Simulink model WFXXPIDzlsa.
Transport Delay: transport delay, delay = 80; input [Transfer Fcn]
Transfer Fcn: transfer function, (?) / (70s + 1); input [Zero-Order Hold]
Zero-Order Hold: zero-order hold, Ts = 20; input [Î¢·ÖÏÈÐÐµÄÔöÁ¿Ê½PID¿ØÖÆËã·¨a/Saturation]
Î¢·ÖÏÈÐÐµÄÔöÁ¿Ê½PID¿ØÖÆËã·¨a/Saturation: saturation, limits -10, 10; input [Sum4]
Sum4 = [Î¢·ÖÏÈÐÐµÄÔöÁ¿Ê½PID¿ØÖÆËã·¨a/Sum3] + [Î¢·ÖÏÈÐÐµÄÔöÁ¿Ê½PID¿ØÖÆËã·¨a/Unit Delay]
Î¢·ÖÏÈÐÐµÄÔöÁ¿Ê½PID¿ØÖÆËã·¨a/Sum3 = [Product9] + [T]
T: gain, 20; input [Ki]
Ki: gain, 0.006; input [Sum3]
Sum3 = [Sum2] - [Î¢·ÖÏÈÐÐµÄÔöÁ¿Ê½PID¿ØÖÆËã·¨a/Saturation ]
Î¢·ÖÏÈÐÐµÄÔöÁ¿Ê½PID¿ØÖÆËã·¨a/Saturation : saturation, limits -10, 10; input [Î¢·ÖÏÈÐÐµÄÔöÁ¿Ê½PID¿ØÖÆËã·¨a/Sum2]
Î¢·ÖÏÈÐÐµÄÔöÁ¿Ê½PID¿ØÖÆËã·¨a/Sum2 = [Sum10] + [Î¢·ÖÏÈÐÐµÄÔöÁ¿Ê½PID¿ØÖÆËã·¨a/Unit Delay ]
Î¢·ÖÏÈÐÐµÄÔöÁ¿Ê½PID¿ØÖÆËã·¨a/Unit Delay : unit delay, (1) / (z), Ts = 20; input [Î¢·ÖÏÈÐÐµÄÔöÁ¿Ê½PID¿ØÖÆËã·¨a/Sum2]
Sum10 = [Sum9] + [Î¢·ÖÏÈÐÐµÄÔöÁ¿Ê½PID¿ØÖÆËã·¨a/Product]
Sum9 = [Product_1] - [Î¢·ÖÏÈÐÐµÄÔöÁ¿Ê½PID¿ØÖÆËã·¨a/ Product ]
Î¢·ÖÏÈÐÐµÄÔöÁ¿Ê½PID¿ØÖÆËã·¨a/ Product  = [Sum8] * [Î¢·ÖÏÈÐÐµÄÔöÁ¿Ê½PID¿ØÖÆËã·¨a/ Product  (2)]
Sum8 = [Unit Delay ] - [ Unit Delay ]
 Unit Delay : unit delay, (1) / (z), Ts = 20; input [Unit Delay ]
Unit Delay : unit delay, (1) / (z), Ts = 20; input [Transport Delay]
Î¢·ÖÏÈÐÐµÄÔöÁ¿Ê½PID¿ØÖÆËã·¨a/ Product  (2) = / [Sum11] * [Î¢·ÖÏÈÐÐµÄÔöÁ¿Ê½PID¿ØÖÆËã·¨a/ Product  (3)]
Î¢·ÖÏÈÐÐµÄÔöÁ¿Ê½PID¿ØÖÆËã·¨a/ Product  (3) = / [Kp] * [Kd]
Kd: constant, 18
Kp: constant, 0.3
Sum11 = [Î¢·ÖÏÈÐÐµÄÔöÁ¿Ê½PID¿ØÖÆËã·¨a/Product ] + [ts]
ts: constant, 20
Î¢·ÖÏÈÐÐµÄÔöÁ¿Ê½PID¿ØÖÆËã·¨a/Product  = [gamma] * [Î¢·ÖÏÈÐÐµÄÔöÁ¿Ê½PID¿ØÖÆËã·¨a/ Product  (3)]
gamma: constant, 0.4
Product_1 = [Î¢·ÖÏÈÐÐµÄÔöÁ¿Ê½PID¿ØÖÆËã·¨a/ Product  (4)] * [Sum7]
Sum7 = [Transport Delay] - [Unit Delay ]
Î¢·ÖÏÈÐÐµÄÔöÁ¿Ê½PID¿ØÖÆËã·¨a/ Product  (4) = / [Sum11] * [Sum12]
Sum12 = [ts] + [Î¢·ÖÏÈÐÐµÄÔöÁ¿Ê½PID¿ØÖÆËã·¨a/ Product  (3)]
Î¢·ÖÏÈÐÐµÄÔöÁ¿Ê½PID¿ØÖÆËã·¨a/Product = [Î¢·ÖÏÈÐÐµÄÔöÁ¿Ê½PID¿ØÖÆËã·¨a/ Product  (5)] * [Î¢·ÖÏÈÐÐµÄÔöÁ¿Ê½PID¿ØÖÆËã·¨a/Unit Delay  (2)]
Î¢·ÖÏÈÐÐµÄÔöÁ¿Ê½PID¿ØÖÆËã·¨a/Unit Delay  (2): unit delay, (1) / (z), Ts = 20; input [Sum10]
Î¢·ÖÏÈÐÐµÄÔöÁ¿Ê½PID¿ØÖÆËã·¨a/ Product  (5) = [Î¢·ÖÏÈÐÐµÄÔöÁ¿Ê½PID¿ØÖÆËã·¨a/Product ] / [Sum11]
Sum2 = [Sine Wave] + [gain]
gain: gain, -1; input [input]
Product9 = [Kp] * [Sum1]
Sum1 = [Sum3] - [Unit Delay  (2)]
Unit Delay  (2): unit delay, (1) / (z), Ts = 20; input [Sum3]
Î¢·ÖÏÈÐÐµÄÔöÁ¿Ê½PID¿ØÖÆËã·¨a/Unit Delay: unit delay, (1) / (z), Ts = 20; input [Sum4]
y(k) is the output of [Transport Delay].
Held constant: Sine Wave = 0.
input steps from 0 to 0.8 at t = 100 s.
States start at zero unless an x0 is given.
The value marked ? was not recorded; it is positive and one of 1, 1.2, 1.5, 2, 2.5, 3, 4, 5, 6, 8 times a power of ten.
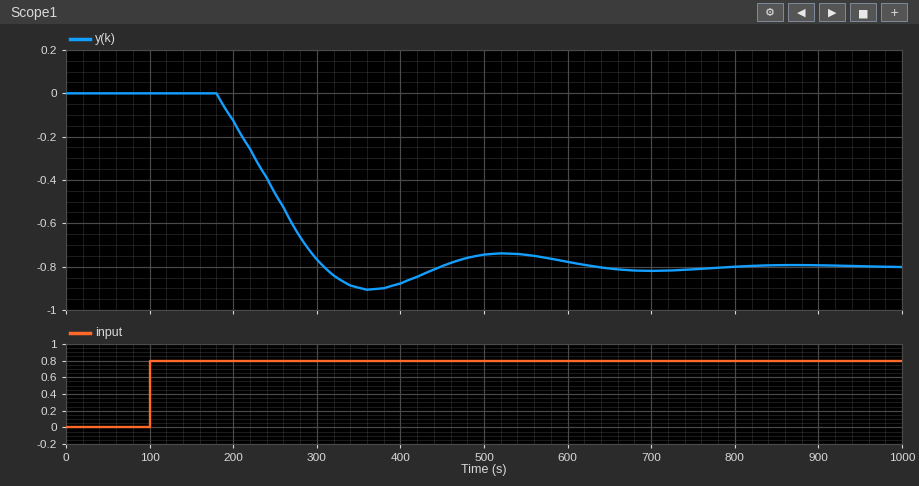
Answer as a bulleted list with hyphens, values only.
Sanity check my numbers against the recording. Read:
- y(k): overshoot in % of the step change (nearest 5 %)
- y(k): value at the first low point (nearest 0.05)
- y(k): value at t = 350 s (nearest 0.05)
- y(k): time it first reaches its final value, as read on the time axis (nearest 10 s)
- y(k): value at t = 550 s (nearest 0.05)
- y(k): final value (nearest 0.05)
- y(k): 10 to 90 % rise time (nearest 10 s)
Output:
- 15 %
- -0.90
- -0.90
- 310 s
- -0.75
- -0.80
- 100 s
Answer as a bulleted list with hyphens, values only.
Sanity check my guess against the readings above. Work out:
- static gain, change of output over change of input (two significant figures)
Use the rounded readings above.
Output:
- -1.0
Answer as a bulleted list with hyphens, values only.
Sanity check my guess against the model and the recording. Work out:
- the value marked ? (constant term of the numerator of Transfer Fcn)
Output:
- 1.5
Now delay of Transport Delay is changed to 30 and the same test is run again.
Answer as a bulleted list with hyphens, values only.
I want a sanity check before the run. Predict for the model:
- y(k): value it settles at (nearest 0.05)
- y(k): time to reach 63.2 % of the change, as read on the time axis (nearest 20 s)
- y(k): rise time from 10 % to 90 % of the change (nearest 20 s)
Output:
- -0.80
- 220 s
- 240 s
